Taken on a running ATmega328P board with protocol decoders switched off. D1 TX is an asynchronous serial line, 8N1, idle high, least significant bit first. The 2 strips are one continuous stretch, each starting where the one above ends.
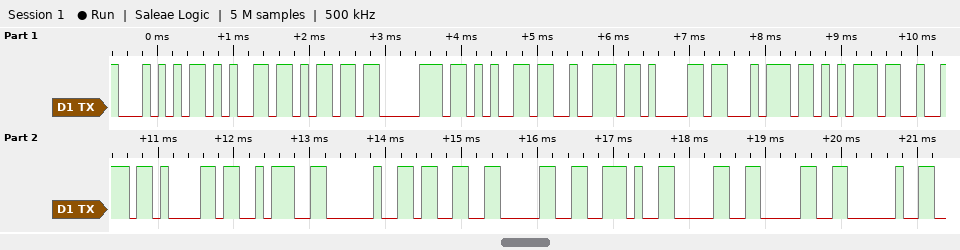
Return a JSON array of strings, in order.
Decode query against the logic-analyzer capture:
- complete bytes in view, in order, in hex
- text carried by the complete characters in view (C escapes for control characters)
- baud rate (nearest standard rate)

["54 65 6D 70 65 72 61 74 75 72 61 3A 20 33 30 2E 30 30 20", "\"Temperatura: 30.00 \"", "9600 baud"]
